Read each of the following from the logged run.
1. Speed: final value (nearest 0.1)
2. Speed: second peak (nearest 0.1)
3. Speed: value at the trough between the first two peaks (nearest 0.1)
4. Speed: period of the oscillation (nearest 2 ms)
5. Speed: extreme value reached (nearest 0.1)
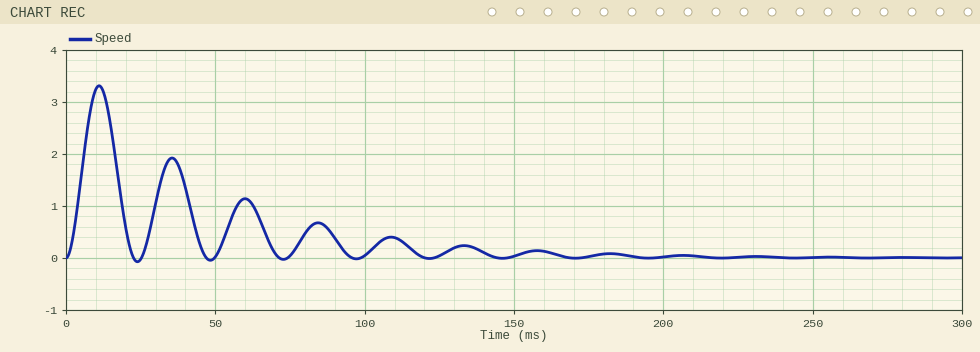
0.0
1.9
-0.1
24 ms
3.3
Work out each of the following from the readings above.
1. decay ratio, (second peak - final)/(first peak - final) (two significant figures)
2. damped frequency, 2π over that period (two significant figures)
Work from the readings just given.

0.58
0.26 rad/ms
